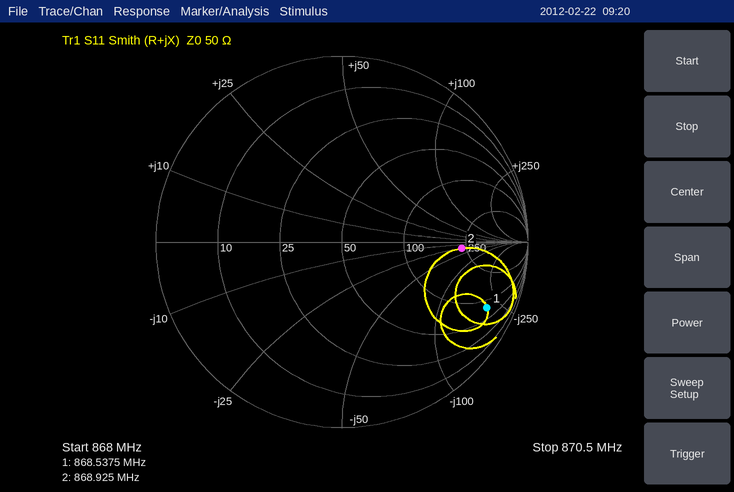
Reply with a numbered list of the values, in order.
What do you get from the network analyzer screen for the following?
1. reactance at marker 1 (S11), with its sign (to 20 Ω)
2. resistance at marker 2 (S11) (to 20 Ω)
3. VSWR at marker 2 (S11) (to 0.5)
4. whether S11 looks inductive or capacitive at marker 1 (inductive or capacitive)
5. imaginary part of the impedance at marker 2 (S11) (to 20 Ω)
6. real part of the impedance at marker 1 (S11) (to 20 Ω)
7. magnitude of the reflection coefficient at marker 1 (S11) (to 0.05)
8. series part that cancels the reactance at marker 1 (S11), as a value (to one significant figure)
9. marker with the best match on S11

1. -200 Ω
2. 220 Ω
3. 4.5
4. capacitive
5. -20 Ω
6. 80 Ω
7. 0.85
8. 40 nH
9. marker 2
